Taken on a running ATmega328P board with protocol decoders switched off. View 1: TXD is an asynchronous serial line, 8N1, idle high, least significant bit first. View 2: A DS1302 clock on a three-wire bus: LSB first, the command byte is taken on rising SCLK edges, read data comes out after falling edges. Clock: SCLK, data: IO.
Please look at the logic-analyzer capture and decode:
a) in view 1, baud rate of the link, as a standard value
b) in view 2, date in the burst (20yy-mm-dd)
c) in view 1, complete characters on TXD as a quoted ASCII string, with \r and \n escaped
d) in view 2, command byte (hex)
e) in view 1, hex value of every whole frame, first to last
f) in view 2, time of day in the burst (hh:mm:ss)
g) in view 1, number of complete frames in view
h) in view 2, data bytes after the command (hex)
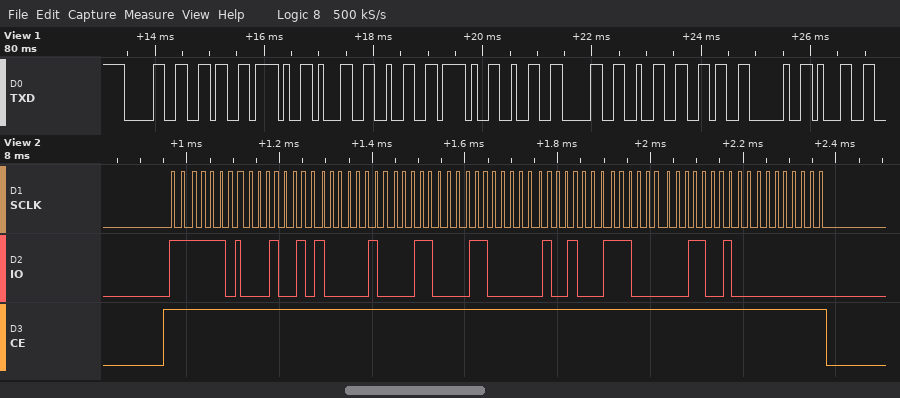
9600 baud
2026-12-06
"06/12/2026 1"
0xBF
30 36 2F 31 32 2F 32 30 32 36 20 31
18:41:48
12
48 41 18 06 12 07 26 00
